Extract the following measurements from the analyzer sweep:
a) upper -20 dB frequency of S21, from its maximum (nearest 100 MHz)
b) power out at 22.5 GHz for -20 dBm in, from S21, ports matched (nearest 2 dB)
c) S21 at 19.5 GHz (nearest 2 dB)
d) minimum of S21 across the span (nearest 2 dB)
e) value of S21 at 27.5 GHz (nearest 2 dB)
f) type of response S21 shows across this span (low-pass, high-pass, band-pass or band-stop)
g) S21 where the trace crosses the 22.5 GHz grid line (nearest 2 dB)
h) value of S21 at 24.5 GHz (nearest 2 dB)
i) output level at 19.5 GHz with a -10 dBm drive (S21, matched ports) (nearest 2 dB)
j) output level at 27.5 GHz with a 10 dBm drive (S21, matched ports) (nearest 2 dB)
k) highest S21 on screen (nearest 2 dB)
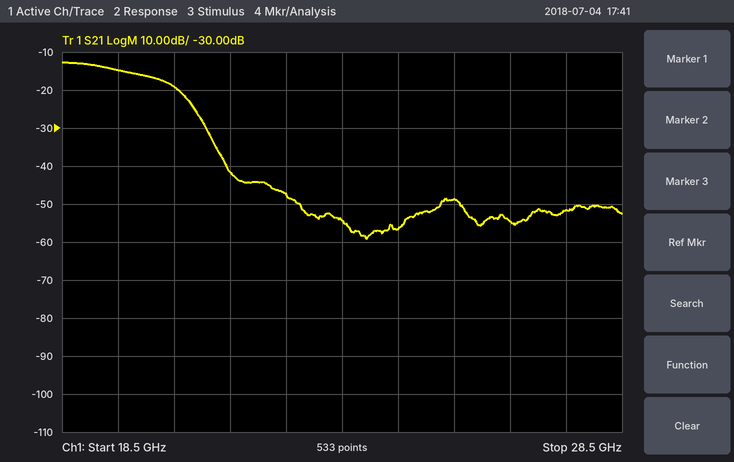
21.2 GHz
-68 dBm
-14 dB
-60 dB
-52 dB
low-pass
-48 dB
-56 dB
-24 dBm
-42 dBm
-12 dB
